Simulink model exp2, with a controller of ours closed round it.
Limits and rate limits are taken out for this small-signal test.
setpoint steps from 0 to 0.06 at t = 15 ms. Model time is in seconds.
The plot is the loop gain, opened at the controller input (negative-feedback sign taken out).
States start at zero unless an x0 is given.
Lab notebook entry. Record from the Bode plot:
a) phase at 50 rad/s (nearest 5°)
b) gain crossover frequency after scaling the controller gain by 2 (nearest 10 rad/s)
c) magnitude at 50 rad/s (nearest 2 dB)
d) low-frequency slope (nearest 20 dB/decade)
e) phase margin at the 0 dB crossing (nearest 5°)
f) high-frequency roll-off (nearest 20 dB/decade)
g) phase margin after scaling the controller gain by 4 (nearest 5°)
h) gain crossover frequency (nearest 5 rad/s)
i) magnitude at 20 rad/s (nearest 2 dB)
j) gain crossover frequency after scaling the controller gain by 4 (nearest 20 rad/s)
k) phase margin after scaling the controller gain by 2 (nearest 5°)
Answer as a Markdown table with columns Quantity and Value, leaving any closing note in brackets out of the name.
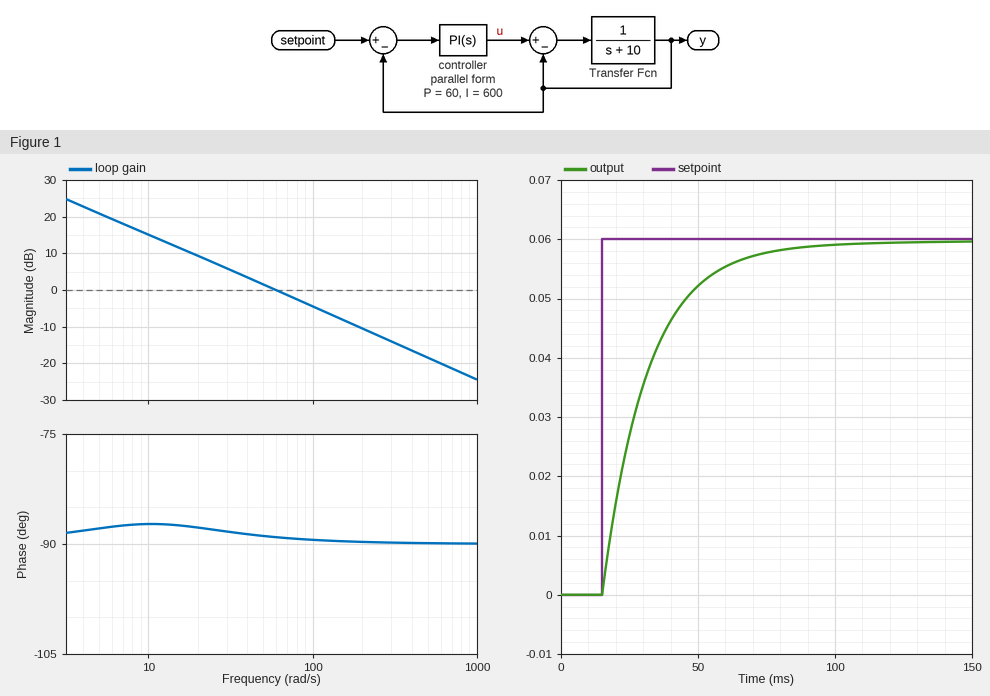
| Quantity | Value |
|---|---|
| phase at 50 rad/s | -90° |
| gain crossover frequency after scaling the controller gain by 2 | 120 rad/s |
| magnitude at 50 rad/s | 2 dB |
| low-frequency slope | -20 dB/decade |
| phase margin at the 0 dB crossing | 90° |
| high-frequency roll-off | -20 dB/decade |
| phase margin after scaling the controller gain by 4 | 90° |
| gain crossover frequency | 60 rad/s |
| magnitude at 20 rad/s | 10 dB |
| gain crossover frequency after scaling the controller gain by 4 | 240 rad/s |
| phase margin after scaling the controller gain by 2 | 90° |
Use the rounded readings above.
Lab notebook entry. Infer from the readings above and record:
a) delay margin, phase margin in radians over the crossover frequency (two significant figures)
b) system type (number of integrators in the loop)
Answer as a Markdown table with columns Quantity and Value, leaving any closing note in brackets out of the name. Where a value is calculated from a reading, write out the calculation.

| Quantity | Value |
|---|---|
| delay margin, phase margin in radians over the crossover frequency | 90 × π / 180 / 60 = 0.026 s |
| system type | 1 |
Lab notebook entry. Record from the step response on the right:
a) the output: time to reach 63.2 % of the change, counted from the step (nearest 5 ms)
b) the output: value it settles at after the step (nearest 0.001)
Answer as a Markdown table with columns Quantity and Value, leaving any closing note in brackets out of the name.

| Quantity | Value |
|---|---|
| the output: time to reach 63.2 % of the change, counted from the step | 15 ms |
| the output: value it settles at after the step | 0.060 |
